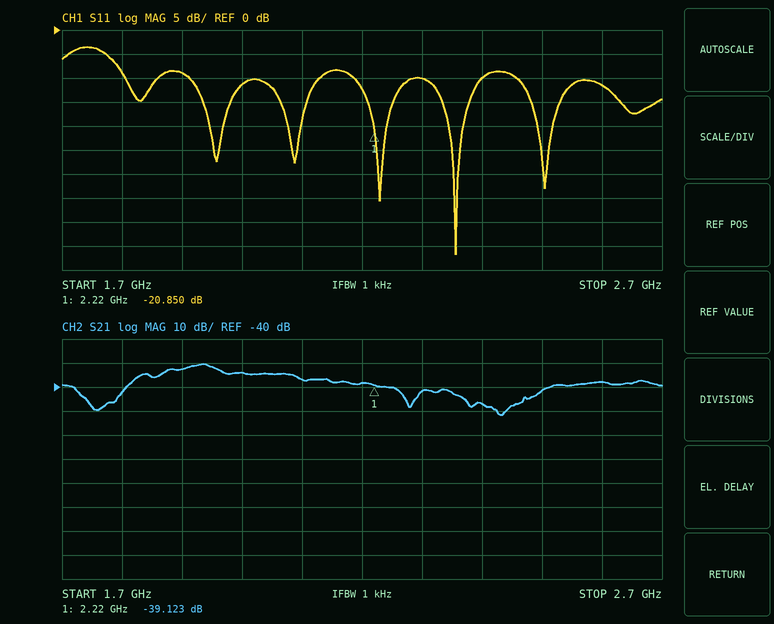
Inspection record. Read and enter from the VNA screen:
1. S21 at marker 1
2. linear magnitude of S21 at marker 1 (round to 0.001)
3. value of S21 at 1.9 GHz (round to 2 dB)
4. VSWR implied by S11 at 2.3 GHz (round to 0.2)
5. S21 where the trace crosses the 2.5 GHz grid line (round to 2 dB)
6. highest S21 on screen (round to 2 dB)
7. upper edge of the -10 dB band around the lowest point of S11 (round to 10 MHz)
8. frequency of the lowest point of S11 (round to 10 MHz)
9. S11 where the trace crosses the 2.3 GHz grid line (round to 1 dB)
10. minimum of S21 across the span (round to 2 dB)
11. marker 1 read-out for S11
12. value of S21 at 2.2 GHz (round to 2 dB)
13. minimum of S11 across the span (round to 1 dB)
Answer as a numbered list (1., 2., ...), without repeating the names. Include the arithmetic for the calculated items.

1. -39.123 dB
2. 10^(-39.123/20) ≈ 0.011
3. -32 dB
4. |Γ| = 10^(-10/20) = 0.3162; VSWR = (1 + 0.3162)/(1 − 0.3162) ≈ 1.92, so 2.0 to the nearest 0.2
5. -42 dB
6. -30 dB
7. 2.40 GHz
8. 2.36 GHz
9. -10 dB
10. -52 dB
11. -20.850 dB
12. -38 dB
13. -47 dB
